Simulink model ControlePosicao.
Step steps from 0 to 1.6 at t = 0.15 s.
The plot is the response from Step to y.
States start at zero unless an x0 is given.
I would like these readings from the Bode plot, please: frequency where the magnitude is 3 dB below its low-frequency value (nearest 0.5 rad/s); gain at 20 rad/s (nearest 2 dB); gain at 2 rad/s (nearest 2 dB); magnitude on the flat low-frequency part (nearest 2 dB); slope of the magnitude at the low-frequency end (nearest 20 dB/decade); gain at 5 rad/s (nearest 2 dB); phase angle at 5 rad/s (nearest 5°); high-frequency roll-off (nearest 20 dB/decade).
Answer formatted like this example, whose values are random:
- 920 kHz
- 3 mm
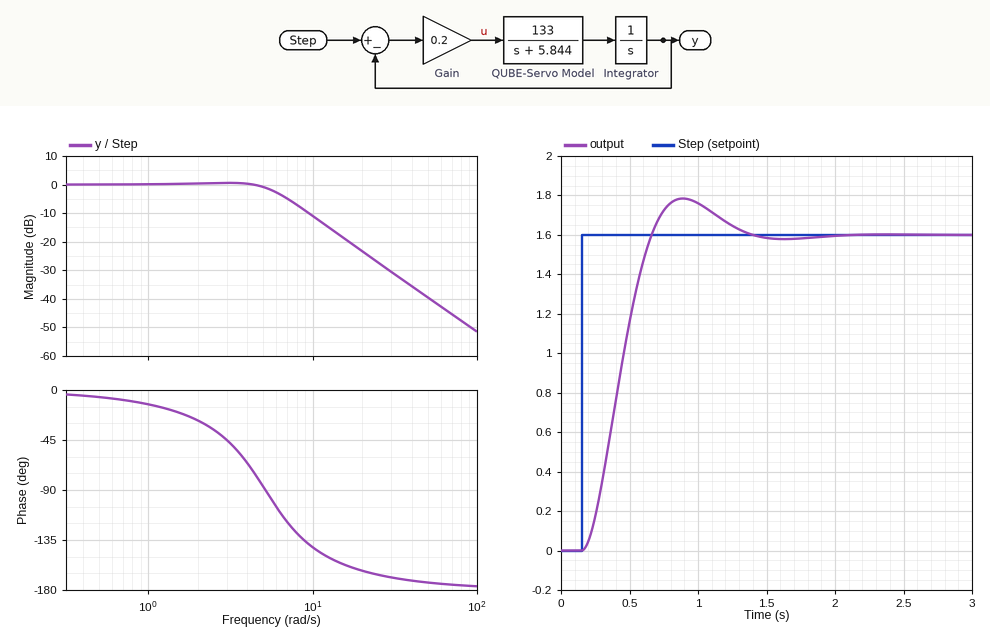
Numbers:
- 6.0 rad/s
- -24 dB
- 0 dB
- 0 dB
- 0 dB/decade
- 0 dB
- -85°
- -40 dB/decade
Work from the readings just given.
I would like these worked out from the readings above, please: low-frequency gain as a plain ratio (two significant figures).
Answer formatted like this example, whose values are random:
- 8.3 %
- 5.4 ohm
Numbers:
- 1.0
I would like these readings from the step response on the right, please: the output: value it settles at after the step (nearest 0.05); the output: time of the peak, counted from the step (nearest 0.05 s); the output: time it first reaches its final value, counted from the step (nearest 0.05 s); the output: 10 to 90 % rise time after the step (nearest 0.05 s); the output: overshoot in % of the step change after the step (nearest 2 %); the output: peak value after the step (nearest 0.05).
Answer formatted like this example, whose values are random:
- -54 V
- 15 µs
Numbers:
- 1.60
- 0.75 s
- 0.50 s
- 0.35 s
- 12 %
- 1.80
